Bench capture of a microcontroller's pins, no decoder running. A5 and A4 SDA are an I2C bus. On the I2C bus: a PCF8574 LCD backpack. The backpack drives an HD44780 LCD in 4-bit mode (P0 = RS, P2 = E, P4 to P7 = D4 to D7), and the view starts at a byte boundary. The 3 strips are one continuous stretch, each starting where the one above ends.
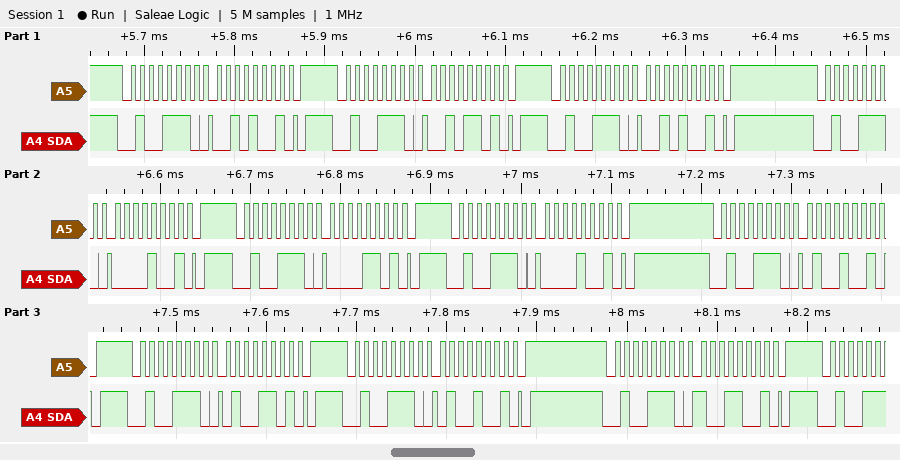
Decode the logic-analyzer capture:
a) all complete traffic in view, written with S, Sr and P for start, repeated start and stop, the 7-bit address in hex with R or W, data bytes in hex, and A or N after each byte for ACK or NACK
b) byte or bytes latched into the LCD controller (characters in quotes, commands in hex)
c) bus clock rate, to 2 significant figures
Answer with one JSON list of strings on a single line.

["S 27W A 29 A P S 27W A 2D A P S 27W A 29 A P S 27W A 09 A P S 27W A 0D A P S 27W A 09 A P S 27W A 49 A P S 27W A 4D A P S 27W A 49 A P S 27W A 99 A P", "' '", "100 kHz"]
